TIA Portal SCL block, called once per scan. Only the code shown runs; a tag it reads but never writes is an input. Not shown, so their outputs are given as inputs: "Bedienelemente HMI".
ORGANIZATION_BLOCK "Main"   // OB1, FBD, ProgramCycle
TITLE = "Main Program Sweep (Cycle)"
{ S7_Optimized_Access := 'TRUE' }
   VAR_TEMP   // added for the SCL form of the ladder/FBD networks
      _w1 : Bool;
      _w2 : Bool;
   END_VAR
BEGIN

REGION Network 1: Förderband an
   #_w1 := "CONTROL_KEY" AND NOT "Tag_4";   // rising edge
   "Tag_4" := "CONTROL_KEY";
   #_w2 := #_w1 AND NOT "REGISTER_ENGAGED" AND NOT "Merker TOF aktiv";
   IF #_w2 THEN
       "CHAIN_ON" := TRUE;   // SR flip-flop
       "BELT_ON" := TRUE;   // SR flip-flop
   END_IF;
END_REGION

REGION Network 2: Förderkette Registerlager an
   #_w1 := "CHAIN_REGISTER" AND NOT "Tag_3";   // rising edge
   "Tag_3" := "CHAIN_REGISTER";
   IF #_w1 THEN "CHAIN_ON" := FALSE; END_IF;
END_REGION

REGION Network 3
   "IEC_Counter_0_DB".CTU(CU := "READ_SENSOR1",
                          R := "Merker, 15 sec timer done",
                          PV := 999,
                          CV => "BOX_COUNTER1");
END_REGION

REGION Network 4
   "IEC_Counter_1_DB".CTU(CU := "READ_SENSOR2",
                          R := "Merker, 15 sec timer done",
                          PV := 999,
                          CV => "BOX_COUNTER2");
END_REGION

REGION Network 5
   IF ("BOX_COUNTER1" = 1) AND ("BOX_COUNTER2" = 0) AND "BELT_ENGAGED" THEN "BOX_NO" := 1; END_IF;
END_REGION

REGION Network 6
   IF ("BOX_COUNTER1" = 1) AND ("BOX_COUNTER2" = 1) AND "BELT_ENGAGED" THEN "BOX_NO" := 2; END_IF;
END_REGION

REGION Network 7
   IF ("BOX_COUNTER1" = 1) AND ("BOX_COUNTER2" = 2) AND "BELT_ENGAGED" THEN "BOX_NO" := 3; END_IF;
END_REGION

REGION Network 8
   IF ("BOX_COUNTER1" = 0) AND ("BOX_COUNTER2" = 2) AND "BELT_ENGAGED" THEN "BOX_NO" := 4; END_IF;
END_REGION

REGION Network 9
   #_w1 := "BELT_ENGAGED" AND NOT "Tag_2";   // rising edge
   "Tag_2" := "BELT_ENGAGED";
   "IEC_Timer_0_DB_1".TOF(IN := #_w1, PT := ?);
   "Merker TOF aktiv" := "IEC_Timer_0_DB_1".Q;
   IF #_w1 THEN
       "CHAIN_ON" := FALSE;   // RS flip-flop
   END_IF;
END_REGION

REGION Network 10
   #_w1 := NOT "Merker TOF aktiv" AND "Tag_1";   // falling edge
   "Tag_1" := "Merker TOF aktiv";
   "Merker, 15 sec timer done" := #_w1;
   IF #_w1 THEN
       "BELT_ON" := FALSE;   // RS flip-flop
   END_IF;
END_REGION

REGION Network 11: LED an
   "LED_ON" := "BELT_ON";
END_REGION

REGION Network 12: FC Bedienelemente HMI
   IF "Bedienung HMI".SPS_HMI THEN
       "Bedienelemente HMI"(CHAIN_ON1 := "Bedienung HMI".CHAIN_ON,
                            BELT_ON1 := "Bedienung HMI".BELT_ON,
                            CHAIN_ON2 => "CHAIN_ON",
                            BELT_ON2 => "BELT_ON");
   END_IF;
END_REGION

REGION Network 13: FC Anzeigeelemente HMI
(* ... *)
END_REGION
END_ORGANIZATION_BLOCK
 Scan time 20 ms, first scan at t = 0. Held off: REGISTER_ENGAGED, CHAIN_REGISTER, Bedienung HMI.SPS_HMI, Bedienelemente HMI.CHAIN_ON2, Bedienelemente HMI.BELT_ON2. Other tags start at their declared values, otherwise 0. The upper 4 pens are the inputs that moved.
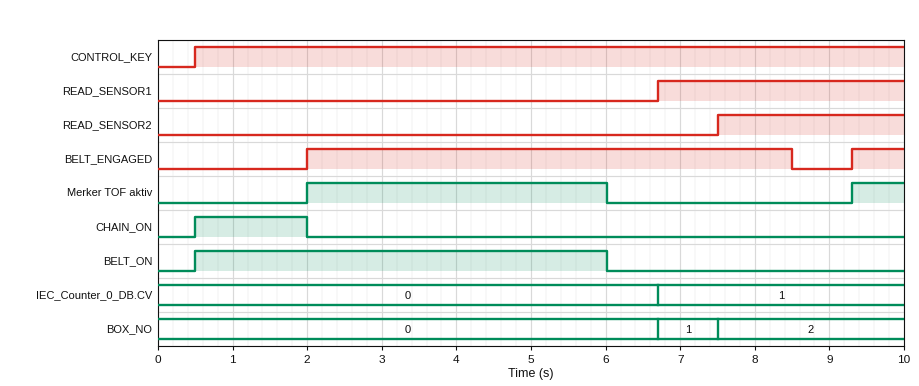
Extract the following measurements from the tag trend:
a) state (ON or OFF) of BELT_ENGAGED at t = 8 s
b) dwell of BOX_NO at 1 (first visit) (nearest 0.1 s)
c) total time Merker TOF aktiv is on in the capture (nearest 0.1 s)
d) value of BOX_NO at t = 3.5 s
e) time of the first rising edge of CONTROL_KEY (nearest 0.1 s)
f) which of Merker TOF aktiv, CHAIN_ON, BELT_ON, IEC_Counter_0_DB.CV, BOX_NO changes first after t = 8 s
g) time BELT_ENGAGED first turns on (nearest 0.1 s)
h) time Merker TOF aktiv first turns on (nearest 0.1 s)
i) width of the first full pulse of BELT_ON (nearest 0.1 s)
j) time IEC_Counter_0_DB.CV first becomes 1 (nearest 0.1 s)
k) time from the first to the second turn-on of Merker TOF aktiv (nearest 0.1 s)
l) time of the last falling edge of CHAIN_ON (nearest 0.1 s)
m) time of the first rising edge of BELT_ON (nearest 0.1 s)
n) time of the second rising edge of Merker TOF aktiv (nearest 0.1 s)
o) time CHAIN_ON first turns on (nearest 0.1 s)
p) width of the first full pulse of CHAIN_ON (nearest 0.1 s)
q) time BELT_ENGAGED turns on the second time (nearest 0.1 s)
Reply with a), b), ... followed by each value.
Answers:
a) ON
b) 0.8 s
c) 4.7 s
d) 0
e) 0.5 s
f) Merker TOF aktiv
g) 2.0 s
h) 2.0 s
i) 5.5 s
j) 6.7 s
k) 7.3 s
l) 2.0 s
m) 0.5 s
n) 9.3 s
o) 0.5 s
p) 1.5 s
q) 9.3 s
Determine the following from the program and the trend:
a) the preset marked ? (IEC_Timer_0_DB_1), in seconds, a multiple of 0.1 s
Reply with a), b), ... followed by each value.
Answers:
a) 4.0 s
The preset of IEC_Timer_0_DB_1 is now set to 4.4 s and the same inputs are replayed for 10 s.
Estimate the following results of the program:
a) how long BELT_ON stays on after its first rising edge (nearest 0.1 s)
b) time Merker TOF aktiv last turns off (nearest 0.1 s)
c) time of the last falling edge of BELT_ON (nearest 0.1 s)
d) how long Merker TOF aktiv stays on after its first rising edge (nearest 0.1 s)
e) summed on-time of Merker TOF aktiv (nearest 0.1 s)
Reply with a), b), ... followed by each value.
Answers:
a) 5.9 s
b) 6.4 s
c) 6.4 s
d) 4.4 s
e) 5.1 s
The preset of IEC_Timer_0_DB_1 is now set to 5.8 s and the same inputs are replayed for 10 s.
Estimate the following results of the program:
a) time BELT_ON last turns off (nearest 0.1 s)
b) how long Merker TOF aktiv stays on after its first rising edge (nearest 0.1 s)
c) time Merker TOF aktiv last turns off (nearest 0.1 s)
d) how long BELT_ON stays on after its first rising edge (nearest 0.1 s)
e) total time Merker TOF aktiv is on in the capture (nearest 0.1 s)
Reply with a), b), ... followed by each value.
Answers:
a) 7.8 s
b) 5.8 s
c) 7.8 s
d) 7.3 s
e) 6.5 s
